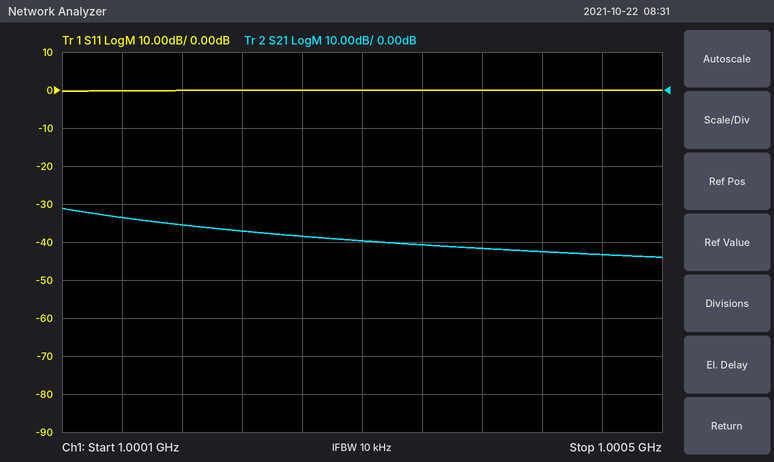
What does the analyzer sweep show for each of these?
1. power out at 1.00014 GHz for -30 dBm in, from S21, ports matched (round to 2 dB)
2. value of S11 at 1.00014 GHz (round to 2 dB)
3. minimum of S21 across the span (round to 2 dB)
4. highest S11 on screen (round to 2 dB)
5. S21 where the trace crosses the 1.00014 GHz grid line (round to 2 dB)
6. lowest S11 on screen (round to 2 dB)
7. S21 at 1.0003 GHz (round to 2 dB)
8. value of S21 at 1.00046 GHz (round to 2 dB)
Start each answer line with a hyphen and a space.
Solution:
- -64 dBm
- 0 dB
- -44 dB
- 0 dB
- -34 dB
- 0 dB
- -40 dB
- -44 dB
